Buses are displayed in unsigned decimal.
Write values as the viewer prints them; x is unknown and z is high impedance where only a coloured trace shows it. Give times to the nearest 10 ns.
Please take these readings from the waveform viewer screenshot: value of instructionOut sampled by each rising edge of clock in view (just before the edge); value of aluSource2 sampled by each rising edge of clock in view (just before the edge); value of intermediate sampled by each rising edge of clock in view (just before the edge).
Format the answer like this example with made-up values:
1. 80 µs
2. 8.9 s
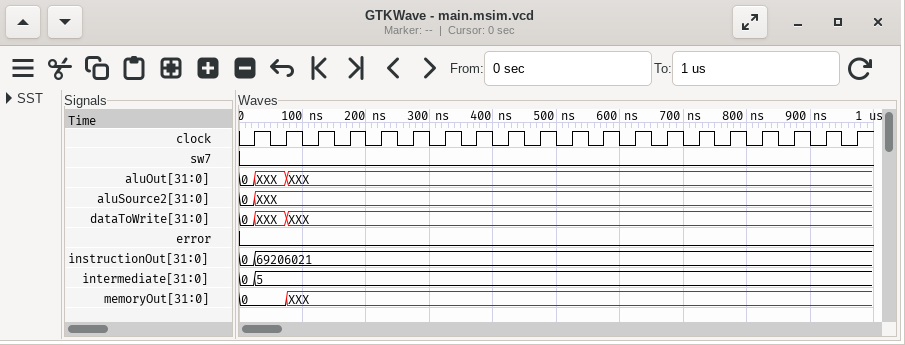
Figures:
1. 0, 69206021, 69206021, 69206021, 69206021, 69206021, 69206021, 69206021, 69206021, 69206021, 69206021, 69206021, 69206021, 69206021, 69206021, 69206021, 69206021, 69206021, 69206021, 69206021
2. 0, XXX, XXX, XXX, XXX, XXX, XXX, XXX, XXX, XXX, XXX, XXX, XXX, XXX, XXX, XXX, XXX, XXX, XXX, XXX
3. 0, 5, 5, 5, 5, 5, 5, 5, 5, 5, 5, 5, 5, 5, 5, 5, 5, 5, 5, 5
